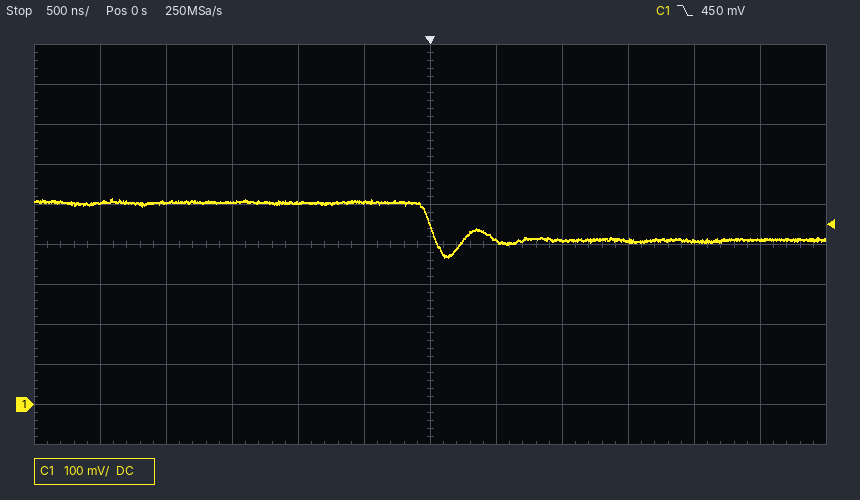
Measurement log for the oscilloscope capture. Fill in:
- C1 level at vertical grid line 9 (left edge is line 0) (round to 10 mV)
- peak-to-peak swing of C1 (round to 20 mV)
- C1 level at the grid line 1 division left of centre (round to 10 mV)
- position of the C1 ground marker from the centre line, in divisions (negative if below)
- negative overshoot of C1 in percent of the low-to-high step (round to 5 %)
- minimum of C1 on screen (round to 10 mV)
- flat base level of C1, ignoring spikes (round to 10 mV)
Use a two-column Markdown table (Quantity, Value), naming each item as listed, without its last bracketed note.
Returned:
| Quantity | Value |
|---|---|
| C1 level at vertical grid line 9 (left edge is line 0) | 410 mV |
| peak-to-peak swing of C1 | 140 mV |
| C1 level at the grid line 1 division left of centre | 510 mV |
| position of the C1 ground marker from the centre line, in divisions | -4.0 div |
| negative overshoot of C1 in percent of the low-to-high step | 45 % |
| minimum of C1 on screen | 370 mV |
| flat base level of C1, ignoring spikes | 410 mV |
